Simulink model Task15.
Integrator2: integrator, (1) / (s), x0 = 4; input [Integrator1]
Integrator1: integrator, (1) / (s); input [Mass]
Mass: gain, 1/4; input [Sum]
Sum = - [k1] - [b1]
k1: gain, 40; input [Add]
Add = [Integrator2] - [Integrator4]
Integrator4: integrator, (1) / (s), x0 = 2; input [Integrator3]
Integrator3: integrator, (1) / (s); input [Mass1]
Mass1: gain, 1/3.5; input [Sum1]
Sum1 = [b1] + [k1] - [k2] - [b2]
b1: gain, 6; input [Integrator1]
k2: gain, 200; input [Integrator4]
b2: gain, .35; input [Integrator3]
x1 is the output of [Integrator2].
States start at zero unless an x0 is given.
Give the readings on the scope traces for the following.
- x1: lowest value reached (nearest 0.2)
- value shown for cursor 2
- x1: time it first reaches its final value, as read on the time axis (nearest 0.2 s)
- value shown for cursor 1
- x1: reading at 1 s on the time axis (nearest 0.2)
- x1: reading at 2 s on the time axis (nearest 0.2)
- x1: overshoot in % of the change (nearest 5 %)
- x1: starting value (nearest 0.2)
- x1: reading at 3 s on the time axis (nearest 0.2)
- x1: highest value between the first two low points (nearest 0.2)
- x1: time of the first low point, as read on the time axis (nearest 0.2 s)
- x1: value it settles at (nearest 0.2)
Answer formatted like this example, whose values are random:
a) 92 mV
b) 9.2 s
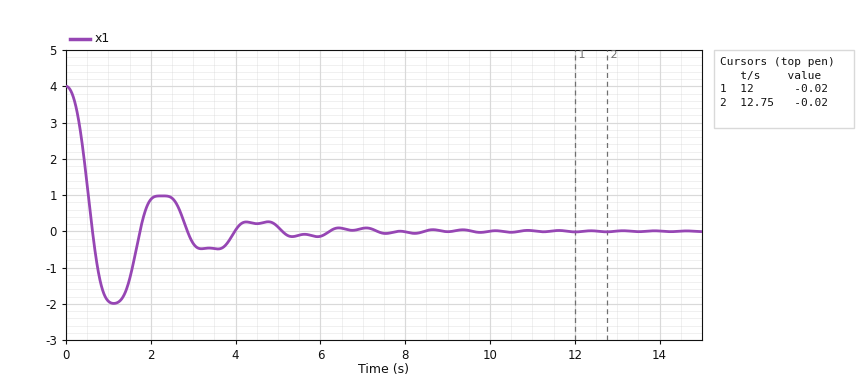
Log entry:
a) -2.0
b) -0.02
c) 0.6 s
d) -0.02
e) -2.0
f) 0.8
g) 50 %
h) 4.0
i) -0.4
j) 1.0
k) 1.2 s
l) 0.0
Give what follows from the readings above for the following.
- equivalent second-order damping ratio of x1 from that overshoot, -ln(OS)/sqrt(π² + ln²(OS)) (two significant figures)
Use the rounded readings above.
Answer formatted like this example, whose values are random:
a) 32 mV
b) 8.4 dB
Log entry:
a) 0.22
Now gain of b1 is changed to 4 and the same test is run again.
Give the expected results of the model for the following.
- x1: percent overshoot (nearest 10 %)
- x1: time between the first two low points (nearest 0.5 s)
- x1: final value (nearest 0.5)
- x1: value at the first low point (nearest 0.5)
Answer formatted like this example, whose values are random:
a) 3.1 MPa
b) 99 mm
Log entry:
a) 60 %
b) 2.0 s
c) 0.0
d) -2.5
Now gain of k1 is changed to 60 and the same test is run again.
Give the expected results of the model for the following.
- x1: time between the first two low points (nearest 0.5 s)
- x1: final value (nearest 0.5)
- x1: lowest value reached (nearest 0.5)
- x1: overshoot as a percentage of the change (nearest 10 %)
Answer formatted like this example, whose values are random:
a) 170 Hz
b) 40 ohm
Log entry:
a) 2.0 s
b) 0.0
c) -2.5
d) 60 %
